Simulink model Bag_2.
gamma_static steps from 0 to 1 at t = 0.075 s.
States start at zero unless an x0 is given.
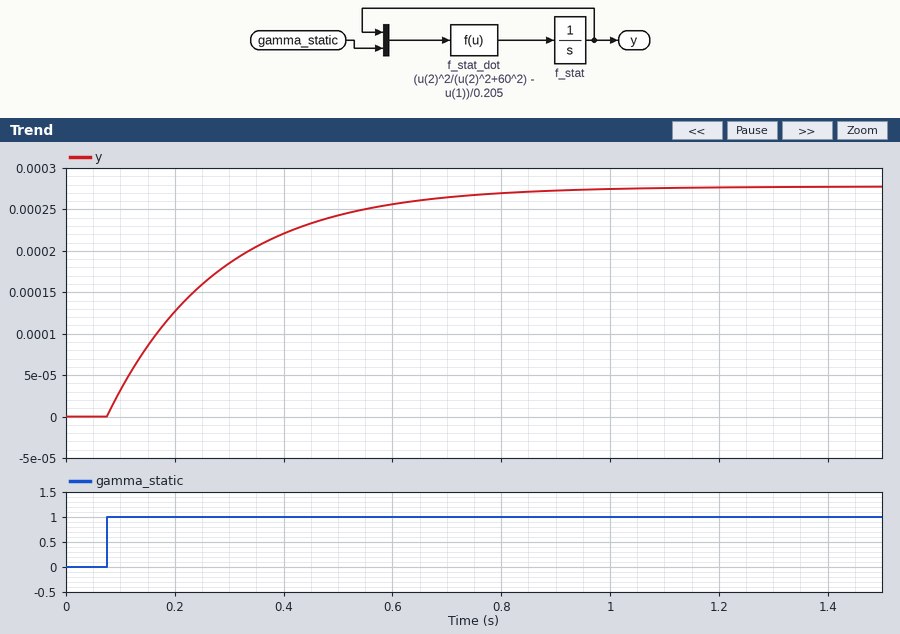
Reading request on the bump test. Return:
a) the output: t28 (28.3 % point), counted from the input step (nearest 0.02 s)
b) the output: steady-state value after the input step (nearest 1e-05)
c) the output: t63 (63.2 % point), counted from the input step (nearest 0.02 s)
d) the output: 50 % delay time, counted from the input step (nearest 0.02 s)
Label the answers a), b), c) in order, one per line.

a) 0.06 s
b) 0.00028
c) 0.20 s
d) 0.14 s
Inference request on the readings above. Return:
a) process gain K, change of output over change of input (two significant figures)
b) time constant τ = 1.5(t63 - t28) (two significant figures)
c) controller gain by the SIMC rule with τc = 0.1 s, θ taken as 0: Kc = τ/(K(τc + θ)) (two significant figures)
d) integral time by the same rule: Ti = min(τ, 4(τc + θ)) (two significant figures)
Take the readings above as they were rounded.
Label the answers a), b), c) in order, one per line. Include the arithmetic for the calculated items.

a) (0.00028 - 0) / 1 = 0.00028
b) 1.5 × (0.2 - 0.06) = 0.21 s
c) 0.21 / (0.00028 × (0.1 + 0)) = 7500
d) min(0.21, 4 × (0.1 + 0)) = 0.21 s
